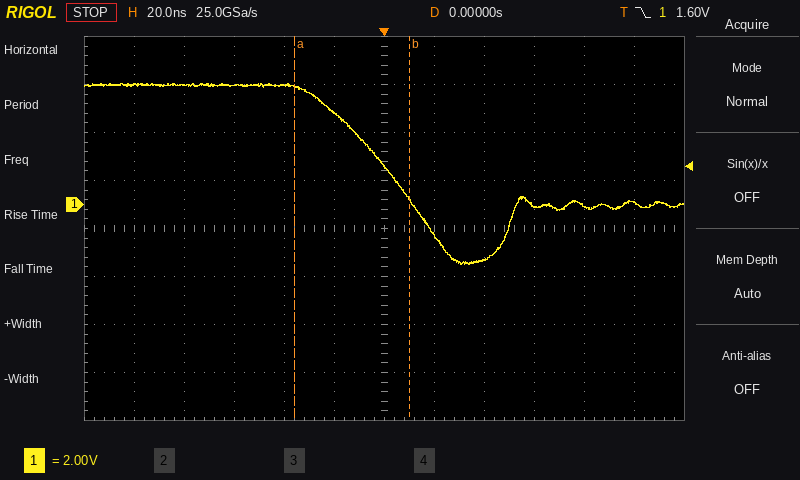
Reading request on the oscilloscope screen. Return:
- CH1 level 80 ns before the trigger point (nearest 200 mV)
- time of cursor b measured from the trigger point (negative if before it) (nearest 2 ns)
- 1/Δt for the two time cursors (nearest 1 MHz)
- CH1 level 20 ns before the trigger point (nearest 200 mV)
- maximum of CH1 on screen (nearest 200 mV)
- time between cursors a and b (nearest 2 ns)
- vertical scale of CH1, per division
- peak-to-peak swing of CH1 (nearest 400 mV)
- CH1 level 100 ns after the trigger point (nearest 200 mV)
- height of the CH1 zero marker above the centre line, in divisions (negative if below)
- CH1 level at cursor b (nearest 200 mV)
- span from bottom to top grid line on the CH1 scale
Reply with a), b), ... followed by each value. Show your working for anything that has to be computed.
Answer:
a) 5.0 V
b) +10 ns
c) 1 / 46 ns ≈ 22 MHz
d) 3.8 V
e) 5.0 V
f) 46 ns
g) 2 V
h) 7.6 V
i) 0.0 V
j) +0.5 div
k) 200 mV
l) 16 V
